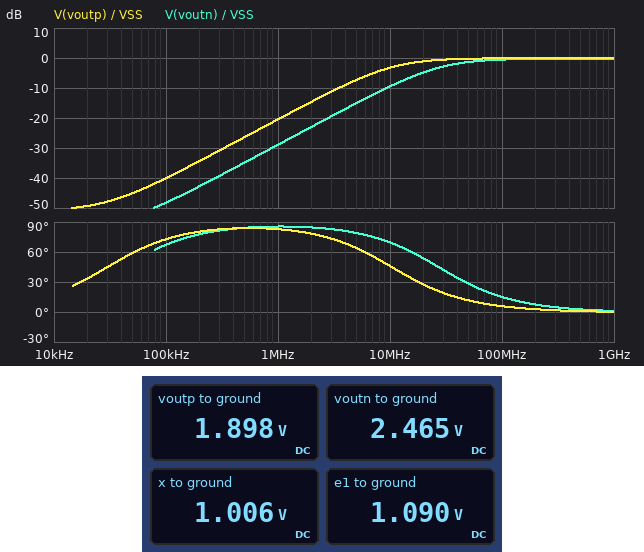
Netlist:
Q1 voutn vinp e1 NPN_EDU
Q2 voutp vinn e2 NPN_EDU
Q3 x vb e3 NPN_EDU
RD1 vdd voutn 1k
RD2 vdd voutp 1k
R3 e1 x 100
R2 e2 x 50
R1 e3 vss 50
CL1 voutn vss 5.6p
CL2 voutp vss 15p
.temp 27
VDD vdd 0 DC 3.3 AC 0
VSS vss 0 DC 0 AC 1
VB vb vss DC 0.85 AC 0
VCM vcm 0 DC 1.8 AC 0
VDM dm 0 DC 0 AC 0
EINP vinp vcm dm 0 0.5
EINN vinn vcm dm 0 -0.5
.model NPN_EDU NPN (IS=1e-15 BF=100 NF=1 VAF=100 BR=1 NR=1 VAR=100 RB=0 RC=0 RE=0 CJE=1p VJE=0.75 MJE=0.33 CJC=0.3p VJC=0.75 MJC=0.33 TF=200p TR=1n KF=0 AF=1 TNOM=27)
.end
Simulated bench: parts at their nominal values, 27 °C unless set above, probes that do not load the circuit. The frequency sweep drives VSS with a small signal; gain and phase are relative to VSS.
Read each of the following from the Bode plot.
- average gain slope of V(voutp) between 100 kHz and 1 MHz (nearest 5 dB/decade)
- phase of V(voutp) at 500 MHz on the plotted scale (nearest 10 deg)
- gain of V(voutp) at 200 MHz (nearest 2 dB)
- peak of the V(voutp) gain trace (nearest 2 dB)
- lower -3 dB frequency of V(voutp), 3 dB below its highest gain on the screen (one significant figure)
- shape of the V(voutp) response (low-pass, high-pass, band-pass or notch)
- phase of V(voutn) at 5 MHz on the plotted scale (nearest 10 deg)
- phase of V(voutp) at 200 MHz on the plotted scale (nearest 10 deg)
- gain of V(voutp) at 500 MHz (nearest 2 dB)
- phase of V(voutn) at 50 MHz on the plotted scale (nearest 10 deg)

20 dB/decade
0 deg
0 dB
0 dB
10 MHz
high-pass
80 deg
0 deg
0 dB
30 deg
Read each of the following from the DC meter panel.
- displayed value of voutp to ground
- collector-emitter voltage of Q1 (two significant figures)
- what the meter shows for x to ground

1.898 V
1.4 V
1.006 V
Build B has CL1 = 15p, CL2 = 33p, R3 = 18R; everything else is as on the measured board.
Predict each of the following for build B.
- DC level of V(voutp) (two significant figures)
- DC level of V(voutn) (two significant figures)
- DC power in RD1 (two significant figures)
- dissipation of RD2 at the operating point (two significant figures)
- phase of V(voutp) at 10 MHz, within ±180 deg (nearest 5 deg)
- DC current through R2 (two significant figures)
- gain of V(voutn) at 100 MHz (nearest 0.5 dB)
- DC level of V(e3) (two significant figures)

2.5 V
1.9 V
2.0 mW
650 µW
25 deg
820 µA
0 dB
110 mV
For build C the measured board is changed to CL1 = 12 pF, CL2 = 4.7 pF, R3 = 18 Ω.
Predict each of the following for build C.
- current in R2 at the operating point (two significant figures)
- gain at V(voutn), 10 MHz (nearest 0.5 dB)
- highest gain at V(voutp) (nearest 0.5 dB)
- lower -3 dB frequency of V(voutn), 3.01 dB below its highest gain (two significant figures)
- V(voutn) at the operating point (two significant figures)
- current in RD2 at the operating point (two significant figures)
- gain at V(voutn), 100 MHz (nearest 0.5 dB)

820 µA
-4.5 dB
-0.5 dB
13 MHz
1.9 V
810 µA
0 dB
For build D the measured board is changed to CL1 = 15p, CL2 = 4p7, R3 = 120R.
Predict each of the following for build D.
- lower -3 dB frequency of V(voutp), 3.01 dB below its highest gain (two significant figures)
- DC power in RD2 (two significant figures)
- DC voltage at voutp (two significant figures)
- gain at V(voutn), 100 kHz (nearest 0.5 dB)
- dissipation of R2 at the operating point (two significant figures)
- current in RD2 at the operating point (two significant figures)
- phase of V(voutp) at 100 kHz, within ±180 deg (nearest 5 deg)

31 MHz
2.2 mW
1.8 V
-40.5 dB
110 µW
1.5 mA
45 deg
